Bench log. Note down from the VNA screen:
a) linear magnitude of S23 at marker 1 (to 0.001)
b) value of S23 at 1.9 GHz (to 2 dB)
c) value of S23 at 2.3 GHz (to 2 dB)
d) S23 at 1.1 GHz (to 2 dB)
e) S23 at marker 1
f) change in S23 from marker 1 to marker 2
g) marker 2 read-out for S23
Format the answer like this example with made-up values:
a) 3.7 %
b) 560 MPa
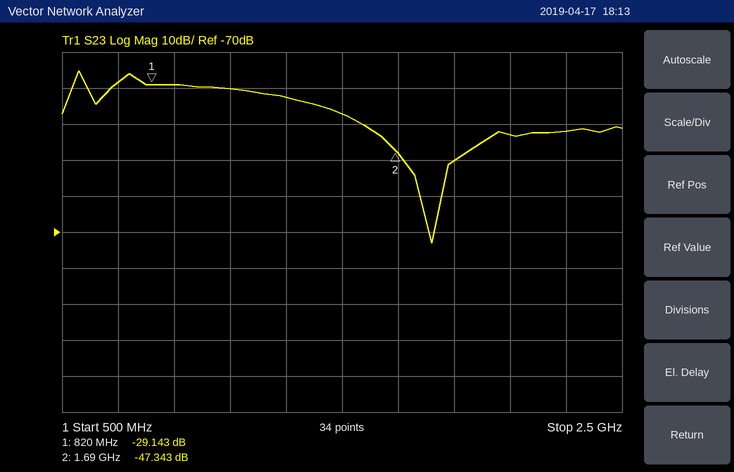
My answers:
a) 0.035
b) -50 dB
c) -42 dB
d) -30 dB
e) -29.143 dB
f) -18.200 dB
g) -47.343 dB
